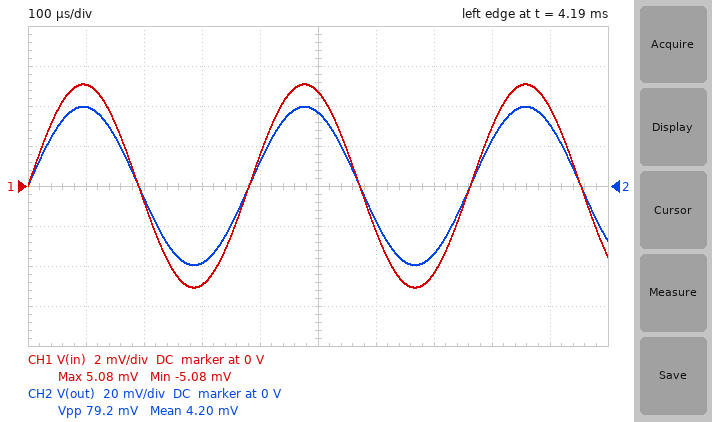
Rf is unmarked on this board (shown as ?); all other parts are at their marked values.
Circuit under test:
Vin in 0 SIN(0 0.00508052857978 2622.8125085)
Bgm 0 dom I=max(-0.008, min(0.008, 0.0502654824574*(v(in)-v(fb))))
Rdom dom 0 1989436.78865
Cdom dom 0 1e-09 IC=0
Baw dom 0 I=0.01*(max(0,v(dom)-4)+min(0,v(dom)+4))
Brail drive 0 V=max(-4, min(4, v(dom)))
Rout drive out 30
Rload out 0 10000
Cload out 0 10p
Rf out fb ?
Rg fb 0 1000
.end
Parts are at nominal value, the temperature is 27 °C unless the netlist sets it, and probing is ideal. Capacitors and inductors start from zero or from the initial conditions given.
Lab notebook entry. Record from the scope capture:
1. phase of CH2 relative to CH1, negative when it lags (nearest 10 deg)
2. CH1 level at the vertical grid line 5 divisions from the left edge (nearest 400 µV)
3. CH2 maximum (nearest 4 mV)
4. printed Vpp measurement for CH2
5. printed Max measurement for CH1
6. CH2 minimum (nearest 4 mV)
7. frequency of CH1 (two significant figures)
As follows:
0 deg
4.8 mV
40 mV
79.2 mV
5.08 mV
-40 mV
2.6 kHz
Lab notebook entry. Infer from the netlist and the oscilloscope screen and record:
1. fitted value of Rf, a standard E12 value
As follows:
6.8 kΩ
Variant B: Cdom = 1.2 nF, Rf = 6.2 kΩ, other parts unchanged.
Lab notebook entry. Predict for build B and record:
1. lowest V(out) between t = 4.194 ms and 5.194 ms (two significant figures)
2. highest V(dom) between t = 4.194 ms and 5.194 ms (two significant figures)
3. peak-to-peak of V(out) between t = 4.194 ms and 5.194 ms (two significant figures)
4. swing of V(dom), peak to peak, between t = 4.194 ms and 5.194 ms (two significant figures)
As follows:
-37 mV
37 mV
73 mV
74 mV
